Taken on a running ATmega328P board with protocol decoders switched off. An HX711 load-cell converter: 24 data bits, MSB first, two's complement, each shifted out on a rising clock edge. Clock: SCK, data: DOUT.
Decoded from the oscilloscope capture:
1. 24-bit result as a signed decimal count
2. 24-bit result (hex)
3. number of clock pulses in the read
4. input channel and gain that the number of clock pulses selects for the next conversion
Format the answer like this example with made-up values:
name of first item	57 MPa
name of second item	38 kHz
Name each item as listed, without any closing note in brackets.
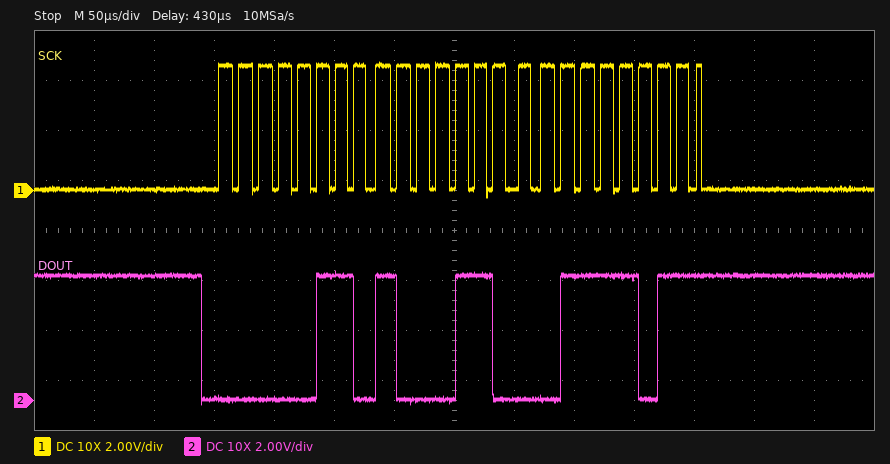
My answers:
24-bit result as a signed decimal count	429179
24-bit result	0x068C7B
number of clock pulses in the read	25
input channel and gain that the number of clock pulses selects for the next conversion	channel A, gain 128
